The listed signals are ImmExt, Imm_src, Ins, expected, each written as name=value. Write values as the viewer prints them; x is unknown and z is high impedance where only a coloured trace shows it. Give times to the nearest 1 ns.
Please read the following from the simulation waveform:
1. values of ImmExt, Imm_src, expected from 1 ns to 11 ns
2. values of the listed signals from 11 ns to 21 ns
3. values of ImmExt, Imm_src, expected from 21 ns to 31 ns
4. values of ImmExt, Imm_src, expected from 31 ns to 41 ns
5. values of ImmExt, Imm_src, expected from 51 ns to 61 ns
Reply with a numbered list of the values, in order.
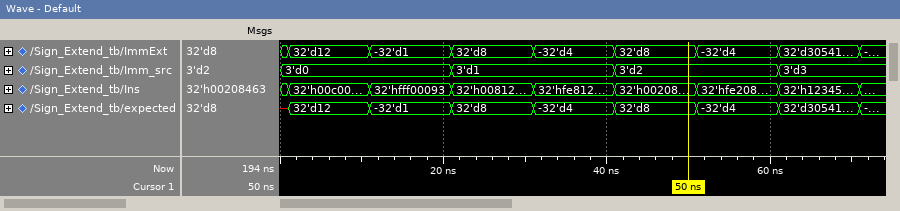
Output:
1. ImmExt=32'd12, Imm_src=3'd0, expected=32'd12
2. ImmExt=-32'd1, Imm_src=3'd0, Ins=32'hfff00093, expected=-32'd1
3. ImmExt=32'd8, Imm_src=3'd1, expected=32'd8
4. ImmExt=-32'd4, Imm_src=3'd1, expected=-32'd4
5. ImmExt=-32'd4, Imm_src=3'd2, expected=-32'd4
